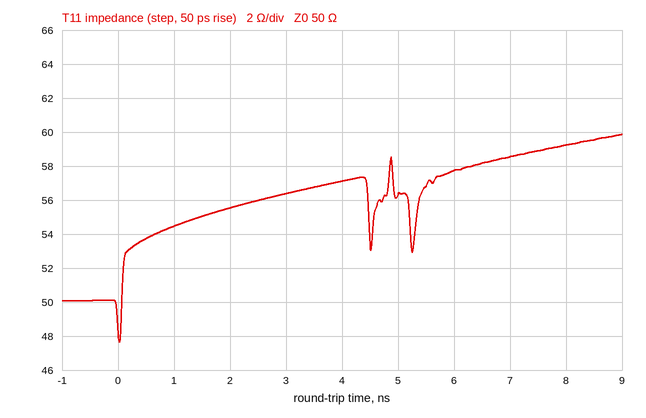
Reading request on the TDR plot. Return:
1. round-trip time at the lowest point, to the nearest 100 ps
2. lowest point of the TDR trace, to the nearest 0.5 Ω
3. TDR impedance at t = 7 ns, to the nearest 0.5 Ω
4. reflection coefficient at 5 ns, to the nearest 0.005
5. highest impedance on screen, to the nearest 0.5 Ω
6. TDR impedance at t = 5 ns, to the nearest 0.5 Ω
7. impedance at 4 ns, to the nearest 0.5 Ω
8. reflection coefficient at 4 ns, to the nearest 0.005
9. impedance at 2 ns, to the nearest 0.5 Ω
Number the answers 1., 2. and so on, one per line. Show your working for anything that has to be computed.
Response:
1. 0.0 ns
2. 47.5 Ω
3. 58.5 Ω
4. (56.5 − 50)/(56.5 + 50) ≈ +0.0610, so +0.060 to the nearest 0.005
5. 60.0 Ω
6. 56.5 Ω
7. 57.0 Ω
8. (57 − 50)/(57 + 50) ≈ +0.065
9. 55.5 Ω
